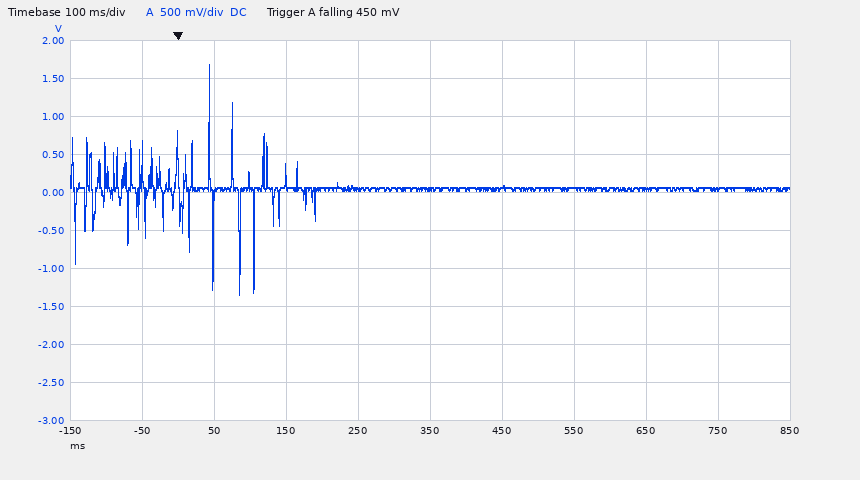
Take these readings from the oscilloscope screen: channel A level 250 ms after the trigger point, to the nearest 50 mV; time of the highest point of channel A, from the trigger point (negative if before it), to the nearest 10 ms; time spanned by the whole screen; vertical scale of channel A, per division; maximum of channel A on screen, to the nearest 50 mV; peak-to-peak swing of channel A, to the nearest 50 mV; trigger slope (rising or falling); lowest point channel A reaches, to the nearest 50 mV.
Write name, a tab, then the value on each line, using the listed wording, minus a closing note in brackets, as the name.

channel A level 250 ms after the trigger point, to the nearest 50 mV	50 mV
time of the highest point of channel A, from the trigger point (negative if before it), to the nearest 10 ms	+40 ms
time spanned by the whole screen	1 s
vertical scale of channel A, per division	500 mV
maximum of channel A on screen, to the nearest 50 mV	1.70 V
peak-to-peak swing of channel A, to the nearest 50 mV	3.05 V
trigger slope	falling
lowest point channel A reaches, to the nearest 50 mV	-1.35 V
